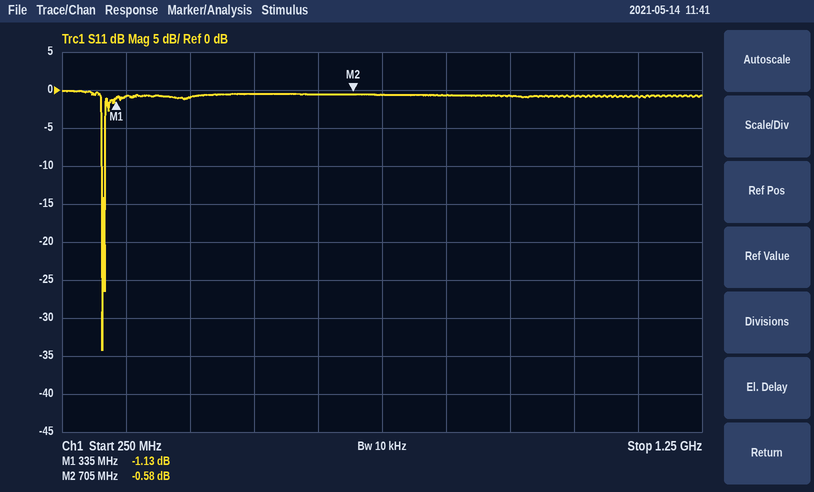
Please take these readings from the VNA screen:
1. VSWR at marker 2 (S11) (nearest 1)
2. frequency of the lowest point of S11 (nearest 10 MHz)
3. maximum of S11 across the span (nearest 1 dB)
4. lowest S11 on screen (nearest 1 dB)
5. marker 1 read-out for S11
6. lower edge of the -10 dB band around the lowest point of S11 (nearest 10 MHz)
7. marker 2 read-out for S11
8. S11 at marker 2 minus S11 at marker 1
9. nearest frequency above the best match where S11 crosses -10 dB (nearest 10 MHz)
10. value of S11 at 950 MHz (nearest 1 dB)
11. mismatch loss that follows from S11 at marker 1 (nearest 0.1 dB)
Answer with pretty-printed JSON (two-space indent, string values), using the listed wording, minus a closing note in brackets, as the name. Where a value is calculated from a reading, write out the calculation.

{
  "VSWR at marker 2 (S11)": "(1 + 0.9354)/(1 − 0.9354) ≈ 30",
  "frequency of the lowest point of S11": "310 MHz",
  "maximum of S11 across the span": "0 dB",
  "lowest S11 on screen": "-34 dB",
  "marker 1 read-out for S11": "-1.13 dB",
  "lower edge of the -10 dB band around the lowest point of S11": "310 MHz",
  "marker 2 read-out for S11": "-0.58 dB",
  "S11 at marker 2 minus S11 at marker 1": "-0.58 − (-1.13) = 0.55 dB",
  "nearest frequency above the best match where S11 crosses -10 dB": "320 MHz",
  "value of S11 at 950 MHz": "-1 dB",
  "mismatch loss that follows from S11 at marker 1": "−10 log10(1 − 10^(-1.13/10)) ≈ 6.4 dB"
}
